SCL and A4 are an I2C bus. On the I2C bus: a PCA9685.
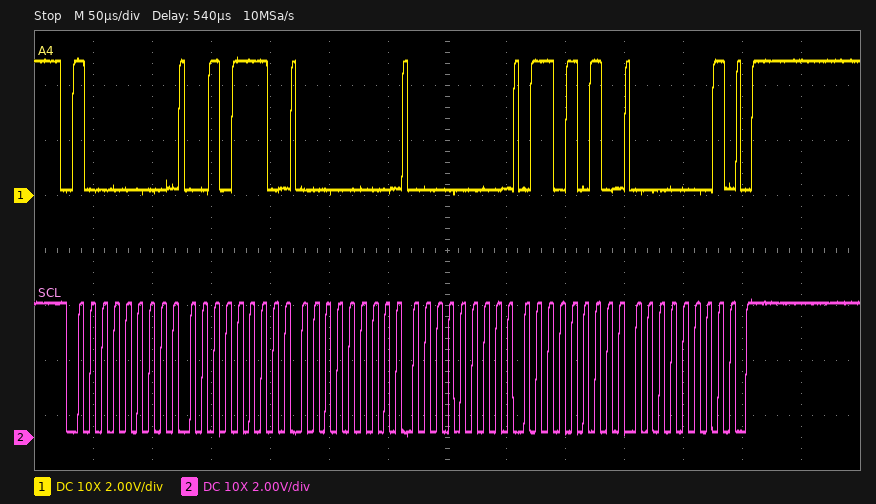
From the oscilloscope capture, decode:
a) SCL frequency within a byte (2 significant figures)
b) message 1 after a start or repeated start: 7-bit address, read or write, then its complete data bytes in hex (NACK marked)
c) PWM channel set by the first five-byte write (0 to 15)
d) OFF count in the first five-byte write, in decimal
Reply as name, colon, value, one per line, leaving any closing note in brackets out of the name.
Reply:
SCL frequency within a byte: 100 kHz
message 1 after a start or repeated start: 7-bit address, read or write, then its complete data bytes in hex: 0x40 write: 2E 00 00 6A 01
PWM channel set by the first five-byte write: 10
OFF count in the first five-byte write, in decimal: 362
